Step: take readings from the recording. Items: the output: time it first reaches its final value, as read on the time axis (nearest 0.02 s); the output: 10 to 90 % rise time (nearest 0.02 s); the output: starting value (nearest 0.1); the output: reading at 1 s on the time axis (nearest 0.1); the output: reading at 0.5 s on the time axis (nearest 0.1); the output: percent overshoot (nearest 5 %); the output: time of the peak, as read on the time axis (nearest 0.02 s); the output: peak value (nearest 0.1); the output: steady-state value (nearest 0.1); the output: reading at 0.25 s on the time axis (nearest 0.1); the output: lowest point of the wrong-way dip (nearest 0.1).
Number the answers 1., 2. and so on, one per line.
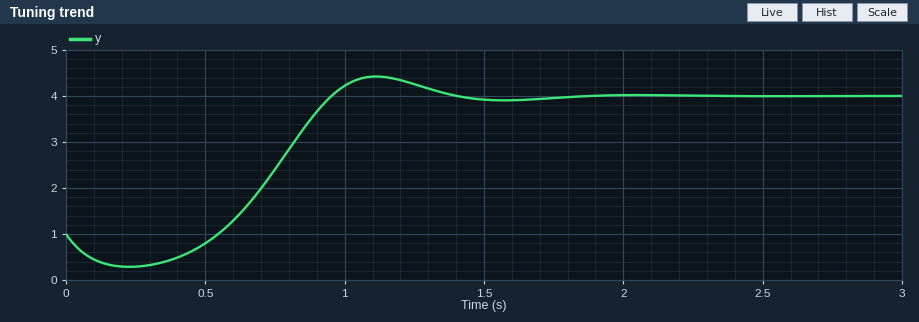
1. 0.96 s
2. 0.30 s
3. 1.0
4. 4.2
5. 0.8
6. 15 %
7. 1.12 s
8. 4.4
9. 4.0
10. 0.3
11. 0.3
